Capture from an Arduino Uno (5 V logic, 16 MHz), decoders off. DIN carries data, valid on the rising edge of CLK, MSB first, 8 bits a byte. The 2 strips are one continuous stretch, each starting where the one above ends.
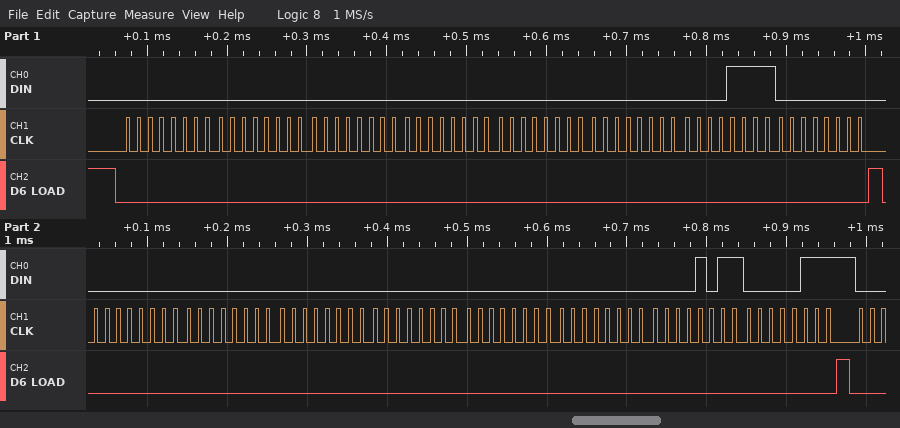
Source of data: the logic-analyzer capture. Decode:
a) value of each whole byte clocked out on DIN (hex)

00 00 00 00 00 00 0F 00 00 00 00 00 00 00 0B 07
